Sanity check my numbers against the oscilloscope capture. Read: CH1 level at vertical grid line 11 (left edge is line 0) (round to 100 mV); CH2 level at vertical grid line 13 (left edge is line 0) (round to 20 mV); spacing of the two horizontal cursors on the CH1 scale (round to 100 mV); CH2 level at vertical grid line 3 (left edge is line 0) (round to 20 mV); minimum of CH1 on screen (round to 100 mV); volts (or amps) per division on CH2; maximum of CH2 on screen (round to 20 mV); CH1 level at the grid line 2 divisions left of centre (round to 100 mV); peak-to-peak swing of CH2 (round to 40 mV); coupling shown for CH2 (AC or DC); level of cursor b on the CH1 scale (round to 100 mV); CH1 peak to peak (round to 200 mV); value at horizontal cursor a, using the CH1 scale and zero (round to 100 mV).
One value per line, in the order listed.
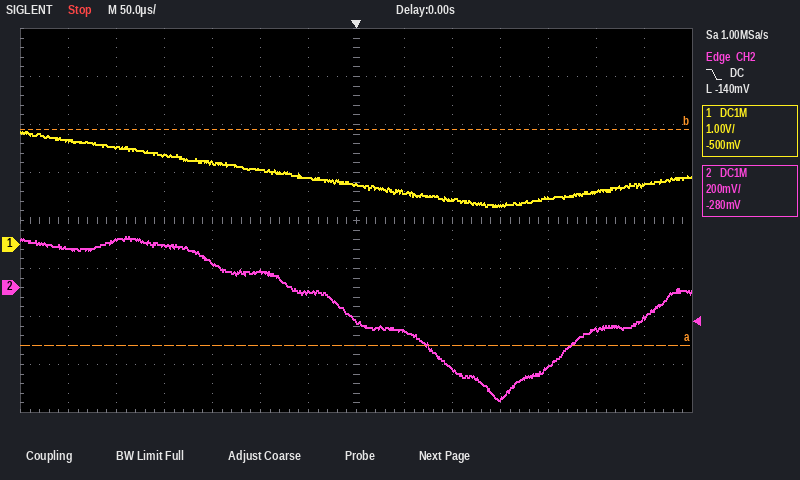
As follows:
1.0 V
-120 mV
4.5 V
180 mV
800 mV
200 mV
220 mV
1.6 V
680 mV
DC
2.4 V
1.6 V
-2.1 V
